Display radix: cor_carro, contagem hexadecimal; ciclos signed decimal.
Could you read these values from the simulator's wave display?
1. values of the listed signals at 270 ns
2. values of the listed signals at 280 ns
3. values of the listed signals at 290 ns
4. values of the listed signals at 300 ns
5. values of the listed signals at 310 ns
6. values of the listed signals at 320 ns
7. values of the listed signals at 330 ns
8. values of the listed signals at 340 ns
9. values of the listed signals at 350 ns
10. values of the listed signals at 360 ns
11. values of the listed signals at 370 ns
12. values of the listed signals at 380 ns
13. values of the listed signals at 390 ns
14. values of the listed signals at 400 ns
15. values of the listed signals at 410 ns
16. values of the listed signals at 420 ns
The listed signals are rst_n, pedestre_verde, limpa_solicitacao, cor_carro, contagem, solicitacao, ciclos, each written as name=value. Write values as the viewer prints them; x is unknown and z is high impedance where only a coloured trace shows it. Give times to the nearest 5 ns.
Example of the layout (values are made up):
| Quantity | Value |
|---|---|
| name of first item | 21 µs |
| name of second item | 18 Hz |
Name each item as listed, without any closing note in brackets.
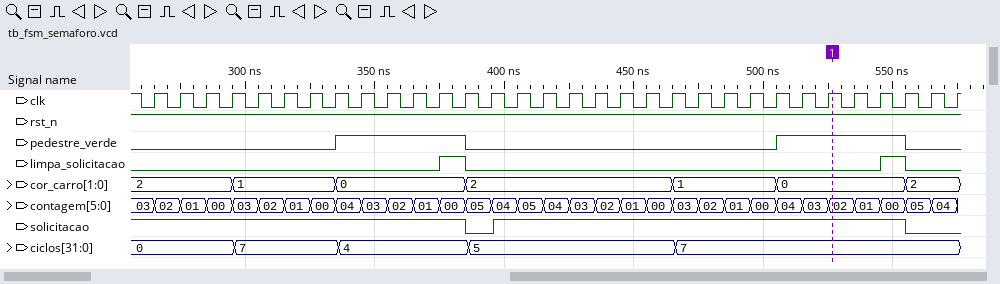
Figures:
| Quantity | Value |
|---|---|
| values of the listed signals at 270 ns | rst_n=1, pedestre_verde=0, limpa_solicitacao=0, cor_carro=2, contagem=02, solicitacao=1, ciclos=0 |
| values of the listed signals at 280 ns | rst_n=1, pedestre_verde=0, limpa_solicitacao=0, cor_carro=2, contagem=01, solicitacao=1, ciclos=0 |
| values of the listed signals at 290 ns | rst_n=1, pedestre_verde=0, limpa_solicitacao=0, cor_carro=2, contagem=00, solicitacao=1, ciclos=0 |
| values of the listed signals at 300 ns | rst_n=1, pedestre_verde=0, limpa_solicitacao=0, cor_carro=1, contagem=03, solicitacao=1, ciclos=7 |
| values of the listed signals at 310 ns | rst_n=1, pedestre_verde=0, limpa_solicitacao=0, cor_carro=1, contagem=02, solicitacao=1, ciclos=7 |
| values of the listed signals at 320 ns | rst_n=1, pedestre_verde=0, limpa_solicitacao=0, cor_carro=1, contagem=01, solicitacao=1, ciclos=7 |
| values of the listed signals at 330 ns | rst_n=1, pedestre_verde=0, limpa_solicitacao=0, cor_carro=1, contagem=00, solicitacao=1, ciclos=7 |
| values of the listed signals at 340 ns | rst_n=1, pedestre_verde=1, limpa_solicitacao=0, cor_carro=0, contagem=04, solicitacao=1, ciclos=4 |
| values of the listed signals at 350 ns | rst_n=1, pedestre_verde=1, limpa_solicitacao=0, cor_carro=0, contagem=03, solicitacao=1, ciclos=4 |
| values of the listed signals at 360 ns | rst_n=1, pedestre_verde=1, limpa_solicitacao=0, cor_carro=0, contagem=02, solicitacao=1, ciclos=4 |
| values of the listed signals at 370 ns | rst_n=1, pedestre_verde=1, limpa_solicitacao=0, cor_carro=0, contagem=01, solicitacao=1, ciclos=4 |
| values of the listed signals at 380 ns | rst_n=1, pedestre_verde=1, limpa_solicitacao=1, cor_carro=0, contagem=00, solicitacao=1, ciclos=4 |
| values of the listed signals at 390 ns | rst_n=1, pedestre_verde=0, limpa_solicitacao=0, cor_carro=2, contagem=05, solicitacao=0, ciclos=5 |
| values of the listed signals at 400 ns | rst_n=1, pedestre_verde=0, limpa_solicitacao=0, cor_carro=2, contagem=04, solicitacao=1, ciclos=5 |
| values of the listed signals at 410 ns | rst_n=1, pedestre_verde=0, limpa_solicitacao=0, cor_carro=2, contagem=05, solicitacao=1, ciclos=5 |
| values of the listed signals at 420 ns | rst_n=1, pedestre_verde=0, limpa_solicitacao=0, cor_carro=2, contagem=04, solicitacao=1, ciclos=5 |
